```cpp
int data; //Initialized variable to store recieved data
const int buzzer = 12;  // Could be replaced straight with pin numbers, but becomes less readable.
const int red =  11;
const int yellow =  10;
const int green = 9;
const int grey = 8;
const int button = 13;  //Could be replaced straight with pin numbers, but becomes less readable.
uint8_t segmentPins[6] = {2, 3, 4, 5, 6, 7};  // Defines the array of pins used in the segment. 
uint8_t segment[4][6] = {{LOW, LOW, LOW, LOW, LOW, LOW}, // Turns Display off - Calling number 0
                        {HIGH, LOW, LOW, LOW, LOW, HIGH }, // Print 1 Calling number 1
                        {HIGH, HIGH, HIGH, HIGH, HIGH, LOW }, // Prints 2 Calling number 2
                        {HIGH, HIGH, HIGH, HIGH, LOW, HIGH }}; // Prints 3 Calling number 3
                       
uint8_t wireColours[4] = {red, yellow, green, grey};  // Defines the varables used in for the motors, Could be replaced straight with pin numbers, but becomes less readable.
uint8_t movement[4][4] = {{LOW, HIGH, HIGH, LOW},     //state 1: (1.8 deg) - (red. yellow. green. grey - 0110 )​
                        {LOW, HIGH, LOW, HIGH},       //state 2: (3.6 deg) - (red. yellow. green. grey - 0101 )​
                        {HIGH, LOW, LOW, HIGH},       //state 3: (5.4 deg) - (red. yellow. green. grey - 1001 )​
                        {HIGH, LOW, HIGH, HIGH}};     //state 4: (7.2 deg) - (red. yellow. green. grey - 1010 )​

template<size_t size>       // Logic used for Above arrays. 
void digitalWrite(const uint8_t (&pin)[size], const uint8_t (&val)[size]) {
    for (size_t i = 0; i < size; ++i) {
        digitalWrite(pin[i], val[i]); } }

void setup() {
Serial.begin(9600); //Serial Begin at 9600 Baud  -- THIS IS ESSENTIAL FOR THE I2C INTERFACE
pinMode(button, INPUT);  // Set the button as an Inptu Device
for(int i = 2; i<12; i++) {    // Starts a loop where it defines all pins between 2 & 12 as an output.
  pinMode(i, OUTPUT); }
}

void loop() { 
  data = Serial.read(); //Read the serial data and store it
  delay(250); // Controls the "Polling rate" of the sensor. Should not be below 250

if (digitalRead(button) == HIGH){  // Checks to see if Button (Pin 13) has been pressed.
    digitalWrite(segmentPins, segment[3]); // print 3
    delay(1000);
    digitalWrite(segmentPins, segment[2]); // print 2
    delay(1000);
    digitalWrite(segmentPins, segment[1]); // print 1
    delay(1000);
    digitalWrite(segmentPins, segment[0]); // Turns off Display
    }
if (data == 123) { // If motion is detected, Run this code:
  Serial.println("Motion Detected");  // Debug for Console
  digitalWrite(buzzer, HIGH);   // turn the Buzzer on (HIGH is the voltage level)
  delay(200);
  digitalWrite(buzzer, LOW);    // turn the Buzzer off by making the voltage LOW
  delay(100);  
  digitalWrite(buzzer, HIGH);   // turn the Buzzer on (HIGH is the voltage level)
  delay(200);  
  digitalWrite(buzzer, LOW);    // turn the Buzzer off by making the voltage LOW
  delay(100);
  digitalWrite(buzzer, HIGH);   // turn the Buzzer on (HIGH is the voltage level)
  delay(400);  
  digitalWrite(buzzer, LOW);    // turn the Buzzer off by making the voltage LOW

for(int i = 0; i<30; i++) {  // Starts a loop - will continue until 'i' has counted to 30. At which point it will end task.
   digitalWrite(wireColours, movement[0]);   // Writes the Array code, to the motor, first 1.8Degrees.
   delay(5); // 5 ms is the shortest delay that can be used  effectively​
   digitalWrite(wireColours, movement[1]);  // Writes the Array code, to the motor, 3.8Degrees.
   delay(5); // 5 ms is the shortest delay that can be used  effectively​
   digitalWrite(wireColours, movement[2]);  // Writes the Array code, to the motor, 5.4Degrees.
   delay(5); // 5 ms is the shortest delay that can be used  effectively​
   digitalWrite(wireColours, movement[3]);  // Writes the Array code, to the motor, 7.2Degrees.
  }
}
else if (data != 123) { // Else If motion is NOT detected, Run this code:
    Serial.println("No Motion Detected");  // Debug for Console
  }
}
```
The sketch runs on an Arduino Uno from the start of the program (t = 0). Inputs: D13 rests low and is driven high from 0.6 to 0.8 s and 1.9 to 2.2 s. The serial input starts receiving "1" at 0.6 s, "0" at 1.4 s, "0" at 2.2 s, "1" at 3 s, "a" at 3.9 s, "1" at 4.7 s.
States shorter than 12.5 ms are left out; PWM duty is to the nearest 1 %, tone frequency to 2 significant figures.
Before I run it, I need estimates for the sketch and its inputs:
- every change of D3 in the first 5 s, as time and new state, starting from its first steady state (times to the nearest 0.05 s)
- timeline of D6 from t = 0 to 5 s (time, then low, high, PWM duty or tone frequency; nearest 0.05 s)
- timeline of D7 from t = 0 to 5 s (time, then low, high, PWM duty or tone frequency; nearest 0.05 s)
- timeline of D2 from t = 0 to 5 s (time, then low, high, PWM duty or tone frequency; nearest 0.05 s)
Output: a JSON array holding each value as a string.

["0 s low; 0.75 s high; 2.75 s low", "0 s low; 1.75 s high; 2.75 s low", "0 s low; 0.75 s high; 1.75 s low; 2.75 s high; 3.75 s low", "0 s low; 0.75 s high; 3.75 s low"]
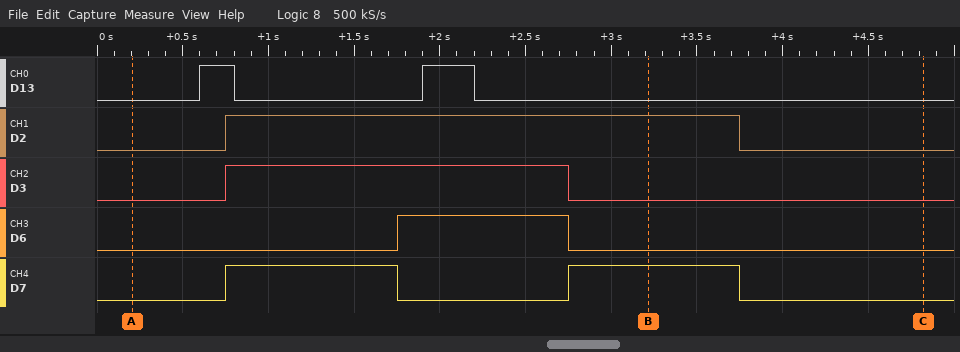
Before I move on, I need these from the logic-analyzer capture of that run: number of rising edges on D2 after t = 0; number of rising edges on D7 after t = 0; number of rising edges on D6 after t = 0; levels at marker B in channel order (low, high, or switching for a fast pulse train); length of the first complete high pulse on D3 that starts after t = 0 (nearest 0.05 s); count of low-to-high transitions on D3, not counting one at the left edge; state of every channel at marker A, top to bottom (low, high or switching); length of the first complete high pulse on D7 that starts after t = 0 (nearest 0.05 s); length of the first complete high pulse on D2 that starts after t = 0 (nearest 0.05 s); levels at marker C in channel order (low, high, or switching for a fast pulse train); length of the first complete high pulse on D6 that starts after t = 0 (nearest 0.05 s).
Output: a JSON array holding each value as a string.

["1", "2", "1", "D13 low, D2 high, D3 low, D6 low, D7 high", "2.00 s", "1", "D13 low, D2 low, D3 low, D6 low, D7 low", "1.00 s", "3.00 s", "D13 low, D2 low, D3 low, D6 low, D7 low", "1.00 s"]
